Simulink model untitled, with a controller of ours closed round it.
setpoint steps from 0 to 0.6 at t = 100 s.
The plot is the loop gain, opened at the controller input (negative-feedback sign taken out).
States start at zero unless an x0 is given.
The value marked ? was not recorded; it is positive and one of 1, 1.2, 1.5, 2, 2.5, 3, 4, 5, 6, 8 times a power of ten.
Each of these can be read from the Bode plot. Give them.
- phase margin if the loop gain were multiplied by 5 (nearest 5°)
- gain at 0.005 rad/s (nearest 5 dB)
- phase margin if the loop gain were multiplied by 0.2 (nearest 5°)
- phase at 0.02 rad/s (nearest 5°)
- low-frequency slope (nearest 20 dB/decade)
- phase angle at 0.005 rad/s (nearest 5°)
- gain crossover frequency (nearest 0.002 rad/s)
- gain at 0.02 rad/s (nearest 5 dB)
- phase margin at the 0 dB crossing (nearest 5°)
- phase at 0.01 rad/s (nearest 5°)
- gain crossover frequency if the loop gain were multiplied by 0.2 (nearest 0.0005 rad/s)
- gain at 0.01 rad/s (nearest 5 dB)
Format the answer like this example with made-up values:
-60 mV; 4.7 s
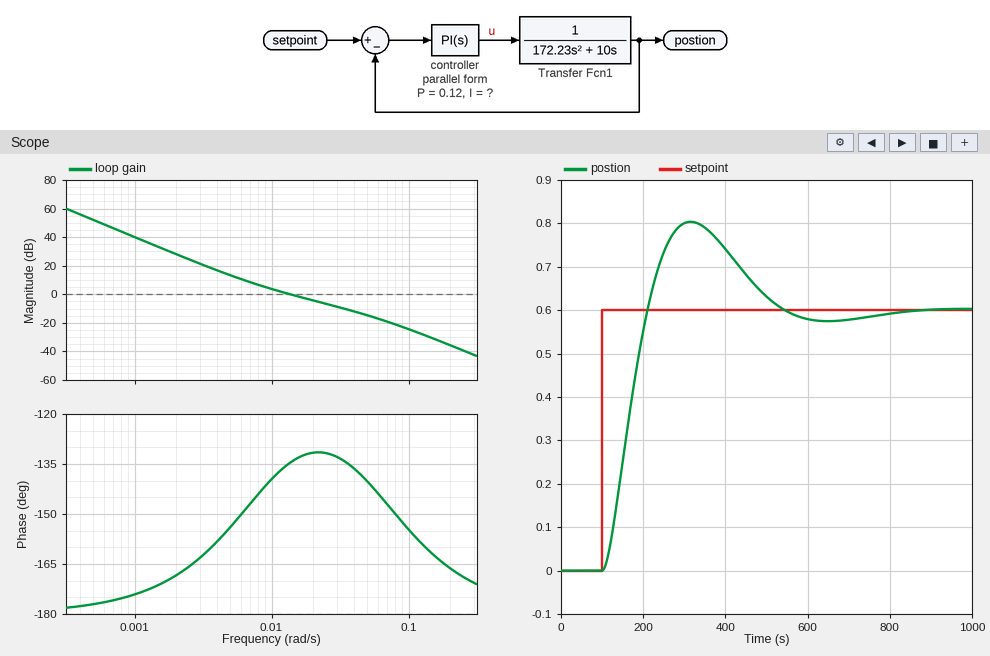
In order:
40°; 15 dB; 25°; -130°; -40 dB/decade; -155°; 0.014 rad/s; -5 dB; 45°; -140°; 0.0050 rad/s; 5 dB
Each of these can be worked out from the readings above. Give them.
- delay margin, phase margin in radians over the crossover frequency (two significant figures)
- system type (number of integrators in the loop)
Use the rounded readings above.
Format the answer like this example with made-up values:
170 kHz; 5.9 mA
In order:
56 s; 2
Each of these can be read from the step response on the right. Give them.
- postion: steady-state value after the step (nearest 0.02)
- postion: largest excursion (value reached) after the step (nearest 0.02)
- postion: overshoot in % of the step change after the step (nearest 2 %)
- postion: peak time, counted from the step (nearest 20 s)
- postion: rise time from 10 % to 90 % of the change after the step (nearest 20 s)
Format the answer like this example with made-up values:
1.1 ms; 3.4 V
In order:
0.60; 0.80; 34 %; 220 s; 80 s
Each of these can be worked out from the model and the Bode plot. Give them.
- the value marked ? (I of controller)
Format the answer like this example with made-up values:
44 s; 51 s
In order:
0.001
